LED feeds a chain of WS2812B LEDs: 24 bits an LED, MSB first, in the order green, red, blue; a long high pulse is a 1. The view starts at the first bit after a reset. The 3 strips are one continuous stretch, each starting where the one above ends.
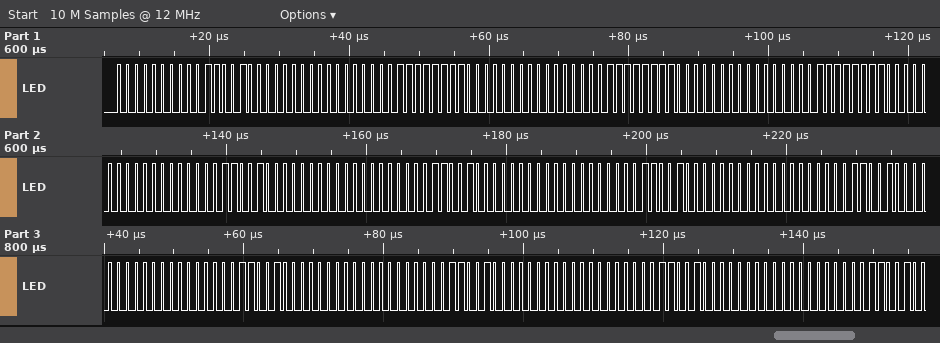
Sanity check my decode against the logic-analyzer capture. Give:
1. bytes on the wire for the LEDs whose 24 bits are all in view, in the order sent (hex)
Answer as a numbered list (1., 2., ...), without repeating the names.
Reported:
1. 00 32 00 00 FF 00 00 FF 00 00 FF 00 00 32 00 00 32 00 00 32 00 00 32 00 00 32 00 00 32 00 00 32 00
